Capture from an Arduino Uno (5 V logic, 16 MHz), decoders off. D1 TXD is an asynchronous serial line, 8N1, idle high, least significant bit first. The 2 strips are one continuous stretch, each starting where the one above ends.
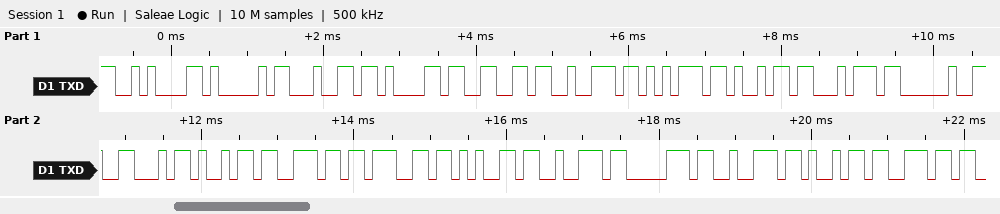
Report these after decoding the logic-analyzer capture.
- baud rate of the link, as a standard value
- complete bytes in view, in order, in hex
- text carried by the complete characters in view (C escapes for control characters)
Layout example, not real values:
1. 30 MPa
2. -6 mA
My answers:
1. 9600 baud
2. 0A 41 64 61 66 72 75 69 74 20 46 69 6E 67 65 72 70 72 69 6E
3. "\nAdafruit Fingerprin"
